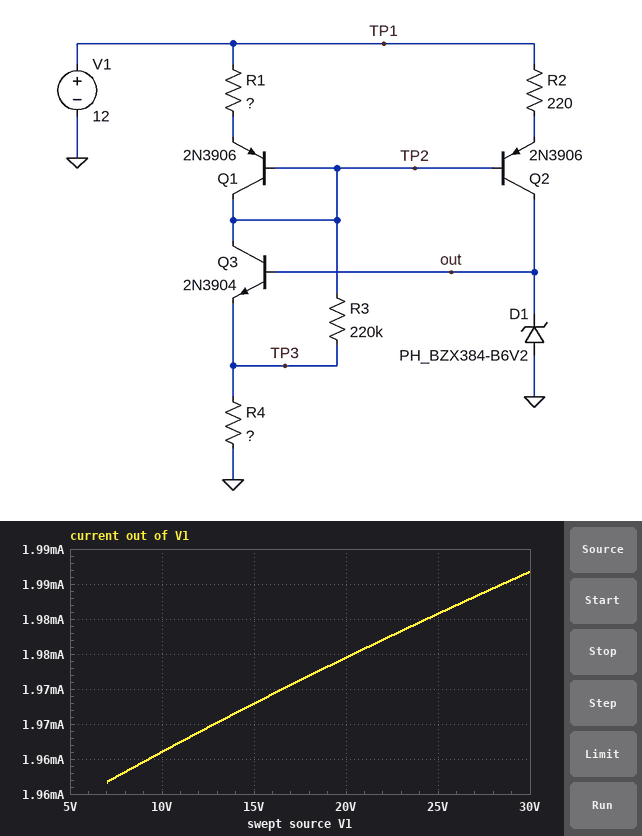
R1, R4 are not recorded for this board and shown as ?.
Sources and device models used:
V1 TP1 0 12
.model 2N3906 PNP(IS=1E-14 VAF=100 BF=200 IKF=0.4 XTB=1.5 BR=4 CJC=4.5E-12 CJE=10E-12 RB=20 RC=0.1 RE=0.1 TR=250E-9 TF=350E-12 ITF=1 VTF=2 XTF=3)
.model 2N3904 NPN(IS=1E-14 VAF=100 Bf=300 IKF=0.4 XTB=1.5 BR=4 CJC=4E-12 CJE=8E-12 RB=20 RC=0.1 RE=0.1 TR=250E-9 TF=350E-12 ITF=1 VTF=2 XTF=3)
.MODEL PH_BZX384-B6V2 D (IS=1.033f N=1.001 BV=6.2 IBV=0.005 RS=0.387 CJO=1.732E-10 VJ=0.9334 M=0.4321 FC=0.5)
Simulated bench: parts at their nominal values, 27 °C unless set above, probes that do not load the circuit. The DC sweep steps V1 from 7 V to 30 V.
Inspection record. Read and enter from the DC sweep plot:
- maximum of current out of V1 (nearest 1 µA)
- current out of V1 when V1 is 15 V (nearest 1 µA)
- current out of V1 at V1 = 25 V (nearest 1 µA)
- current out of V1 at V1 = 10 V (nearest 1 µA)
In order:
1.992 mA
1.973 mA
1.986 mA
1.966 mA
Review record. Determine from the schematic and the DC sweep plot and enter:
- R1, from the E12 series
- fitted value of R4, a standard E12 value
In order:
330 Ω
6.8 kΩ
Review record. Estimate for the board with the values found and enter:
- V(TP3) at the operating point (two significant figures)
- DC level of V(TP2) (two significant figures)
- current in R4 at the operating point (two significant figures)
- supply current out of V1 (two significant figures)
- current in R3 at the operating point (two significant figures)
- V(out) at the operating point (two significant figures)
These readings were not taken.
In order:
5.5 V
11 V
810 µA
2.0 mA
25 µA
6.2 V
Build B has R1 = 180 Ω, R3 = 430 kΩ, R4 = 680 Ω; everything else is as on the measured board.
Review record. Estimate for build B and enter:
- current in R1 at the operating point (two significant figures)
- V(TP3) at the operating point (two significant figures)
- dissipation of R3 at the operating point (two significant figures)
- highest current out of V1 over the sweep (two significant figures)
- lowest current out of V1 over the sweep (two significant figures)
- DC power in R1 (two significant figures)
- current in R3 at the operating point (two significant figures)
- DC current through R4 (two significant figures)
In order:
8.0 mA
5.5 V
44 µW
15 mA
8.7 mA
12 mW
10 µA
8.1 mA
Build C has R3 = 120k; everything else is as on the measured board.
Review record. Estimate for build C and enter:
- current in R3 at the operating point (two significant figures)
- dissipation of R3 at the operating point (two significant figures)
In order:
46 µA
260 µW
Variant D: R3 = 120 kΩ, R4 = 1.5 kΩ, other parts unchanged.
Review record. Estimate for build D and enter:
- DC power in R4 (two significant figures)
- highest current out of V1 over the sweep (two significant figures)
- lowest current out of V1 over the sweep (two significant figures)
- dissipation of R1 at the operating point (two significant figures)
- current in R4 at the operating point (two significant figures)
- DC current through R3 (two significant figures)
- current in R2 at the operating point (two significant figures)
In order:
20 mW
9.1 mA
6.1 mA
4.4 mW
3.7 mA
38 µA
5.4 mA
